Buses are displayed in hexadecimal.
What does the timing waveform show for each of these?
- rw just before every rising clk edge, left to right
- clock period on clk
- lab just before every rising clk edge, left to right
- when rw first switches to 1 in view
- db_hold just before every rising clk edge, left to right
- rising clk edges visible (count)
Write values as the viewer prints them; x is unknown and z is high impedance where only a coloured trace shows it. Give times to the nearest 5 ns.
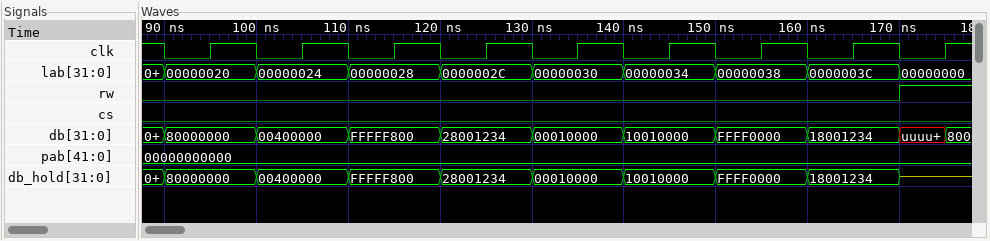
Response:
0 0 0 0 0 0 0 0 1
10 ns
00000020, 00000024, 00000028, 0000002C, 00000030, 00000034, 00000038, 0000003C, 00000000
170 ns
80000000, 00400000, FFFFF800, 28001234, 00010000, 10010000, FFFF0000, 18001234, z
9
